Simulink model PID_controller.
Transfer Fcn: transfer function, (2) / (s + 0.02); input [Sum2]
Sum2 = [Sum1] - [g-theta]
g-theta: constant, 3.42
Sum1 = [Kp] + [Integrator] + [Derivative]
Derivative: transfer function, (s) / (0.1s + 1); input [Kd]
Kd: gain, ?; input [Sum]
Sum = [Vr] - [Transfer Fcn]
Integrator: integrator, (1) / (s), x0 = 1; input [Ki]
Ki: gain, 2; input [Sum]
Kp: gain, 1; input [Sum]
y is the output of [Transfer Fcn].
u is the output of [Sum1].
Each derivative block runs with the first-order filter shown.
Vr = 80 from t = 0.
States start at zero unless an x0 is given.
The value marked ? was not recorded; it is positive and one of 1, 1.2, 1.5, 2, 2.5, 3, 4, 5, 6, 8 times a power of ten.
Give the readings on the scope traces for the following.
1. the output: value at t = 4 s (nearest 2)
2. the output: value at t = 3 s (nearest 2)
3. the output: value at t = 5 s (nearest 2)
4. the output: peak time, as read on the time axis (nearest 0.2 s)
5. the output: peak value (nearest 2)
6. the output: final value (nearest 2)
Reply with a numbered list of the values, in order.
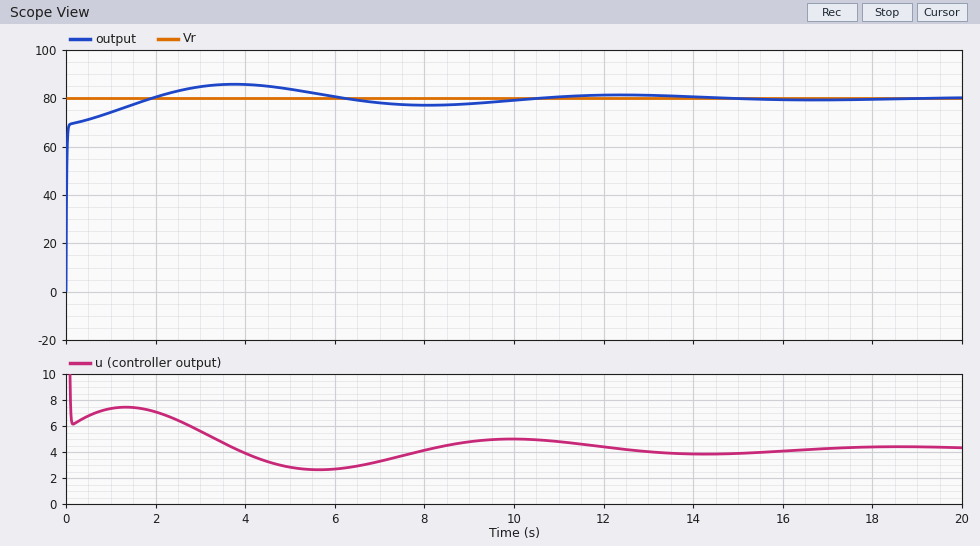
1. 86
2. 84
3. 84
4. 3.8 s
5. 86
6. 80
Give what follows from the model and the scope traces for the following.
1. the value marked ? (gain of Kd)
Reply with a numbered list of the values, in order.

1. 3
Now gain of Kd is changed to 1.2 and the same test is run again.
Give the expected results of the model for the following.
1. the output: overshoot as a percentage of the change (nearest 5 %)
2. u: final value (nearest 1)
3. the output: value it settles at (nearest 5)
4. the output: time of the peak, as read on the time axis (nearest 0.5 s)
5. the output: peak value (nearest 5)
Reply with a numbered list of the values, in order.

1. 10 %
2. 4
3. 80
4. 2.5 s
5. 90
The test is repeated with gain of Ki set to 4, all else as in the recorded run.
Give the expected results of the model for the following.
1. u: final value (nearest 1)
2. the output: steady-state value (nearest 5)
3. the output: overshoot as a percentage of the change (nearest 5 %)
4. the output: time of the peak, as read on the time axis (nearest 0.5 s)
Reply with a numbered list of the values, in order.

1. 4
2. 80
3. 10 %
4. 2.5 s
